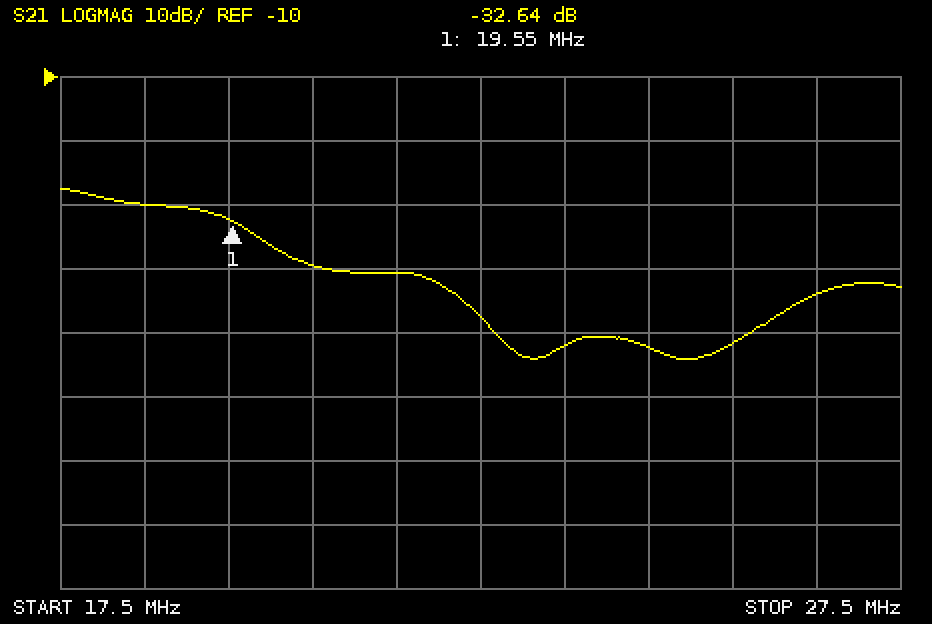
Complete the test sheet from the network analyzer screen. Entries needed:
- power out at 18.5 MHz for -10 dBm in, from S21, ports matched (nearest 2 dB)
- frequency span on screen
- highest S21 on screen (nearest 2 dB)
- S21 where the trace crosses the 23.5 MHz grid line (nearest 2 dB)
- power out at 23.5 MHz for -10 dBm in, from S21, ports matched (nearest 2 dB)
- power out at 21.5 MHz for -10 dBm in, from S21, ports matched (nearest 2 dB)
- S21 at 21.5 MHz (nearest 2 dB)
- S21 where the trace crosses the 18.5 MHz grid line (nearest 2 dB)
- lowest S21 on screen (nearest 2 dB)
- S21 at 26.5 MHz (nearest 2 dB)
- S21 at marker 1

-40 dBm
10 MHz
-28 dB
-52 dB
-62 dBm
-50 dBm
-40 dB
-30 dB
-54 dB
-44 dB
-32.64 dB
